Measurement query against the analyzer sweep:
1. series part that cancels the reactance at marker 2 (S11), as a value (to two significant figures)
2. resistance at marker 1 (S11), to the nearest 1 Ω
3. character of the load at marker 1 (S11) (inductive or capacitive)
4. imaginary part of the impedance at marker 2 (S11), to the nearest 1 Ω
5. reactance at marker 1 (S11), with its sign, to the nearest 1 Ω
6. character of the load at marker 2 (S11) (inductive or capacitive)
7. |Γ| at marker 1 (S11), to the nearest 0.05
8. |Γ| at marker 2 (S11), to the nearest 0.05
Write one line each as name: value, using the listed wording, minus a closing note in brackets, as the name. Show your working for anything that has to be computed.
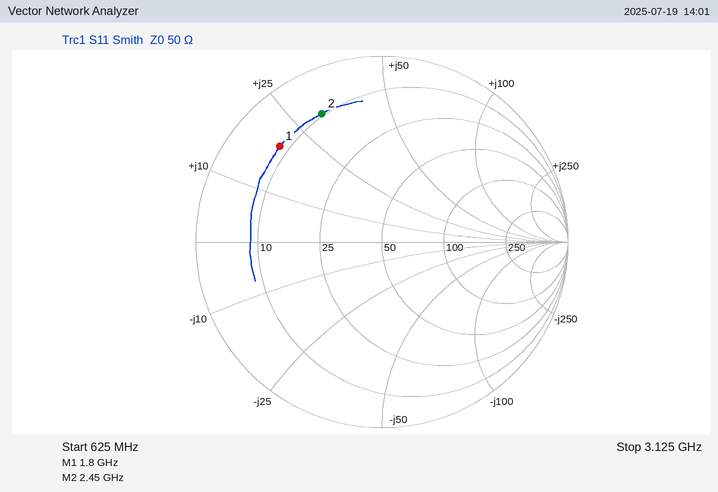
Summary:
series part that cancels the reactance at marker 2 (S11), as a value: C = 1/(2π × 2.45 GHz × 31 Ω) ≈ 2.1 pF
resistance at marker 1 (S11), to the nearest 1 Ω: 8 Ω
character of the load at marker 1 (S11): inductive
imaginary part of the impedance at marker 2 (S11), to the nearest 1 Ω: +31 Ω
reactance at marker 1 (S11), with its sign, to the nearest 1 Ω: +19 Ω
character of the load at marker 2 (S11): inductive
|Γ| at marker 1 (S11), to the nearest 0.05: 0.75
|Γ| at marker 2 (S11), to the nearest 0.05: 0.75
